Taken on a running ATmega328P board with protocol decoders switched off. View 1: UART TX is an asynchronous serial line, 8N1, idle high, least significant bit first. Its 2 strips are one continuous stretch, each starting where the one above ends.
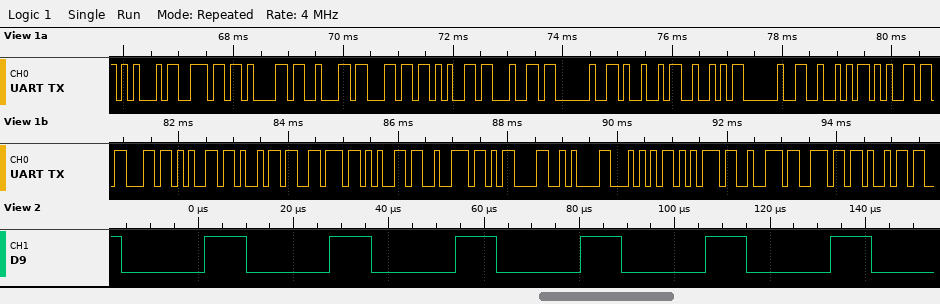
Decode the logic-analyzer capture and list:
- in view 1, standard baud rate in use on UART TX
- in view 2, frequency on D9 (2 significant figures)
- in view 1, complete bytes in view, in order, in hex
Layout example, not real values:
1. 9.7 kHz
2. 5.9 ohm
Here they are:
1. 9600 baud
2. 38 kHz
3. 0x45 0x6E 0x61 0x62 0x6C 0x65 0x64 0x20 0x49 0x52 0x20 0x52 0x65 0x63 0x65 0x69 0x76 0x65 0x72 0x0D 0x0A 0x54 0x75 0x72 0x6E 0x69
